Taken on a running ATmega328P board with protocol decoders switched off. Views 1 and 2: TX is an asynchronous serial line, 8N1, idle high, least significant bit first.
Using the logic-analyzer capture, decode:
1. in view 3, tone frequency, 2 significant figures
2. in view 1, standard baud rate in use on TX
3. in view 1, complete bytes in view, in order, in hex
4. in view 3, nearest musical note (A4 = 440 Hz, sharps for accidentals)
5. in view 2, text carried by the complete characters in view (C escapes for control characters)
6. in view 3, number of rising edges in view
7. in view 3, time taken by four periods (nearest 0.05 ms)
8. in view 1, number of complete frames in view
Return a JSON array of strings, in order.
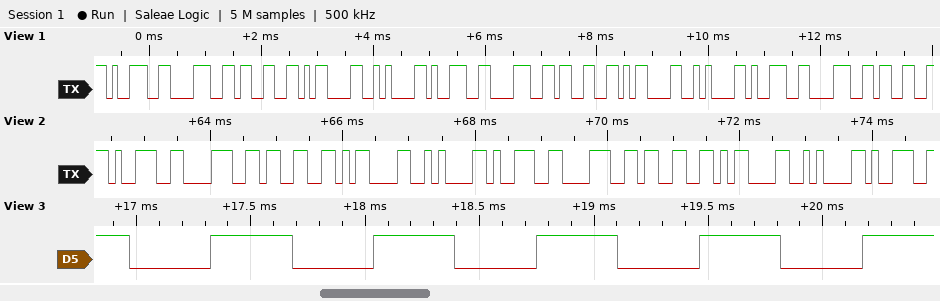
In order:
["1.4 kHz", "9600 baud", "0x39 0x38 0x33 0x0D 0x0A 0x39 0x38 0x33 0x0D 0x0A 0x39 0x38 0x33", "F6", "\"983\\r\\n983\\r\\n9\"", "5", "2.85 ms", "13"]
